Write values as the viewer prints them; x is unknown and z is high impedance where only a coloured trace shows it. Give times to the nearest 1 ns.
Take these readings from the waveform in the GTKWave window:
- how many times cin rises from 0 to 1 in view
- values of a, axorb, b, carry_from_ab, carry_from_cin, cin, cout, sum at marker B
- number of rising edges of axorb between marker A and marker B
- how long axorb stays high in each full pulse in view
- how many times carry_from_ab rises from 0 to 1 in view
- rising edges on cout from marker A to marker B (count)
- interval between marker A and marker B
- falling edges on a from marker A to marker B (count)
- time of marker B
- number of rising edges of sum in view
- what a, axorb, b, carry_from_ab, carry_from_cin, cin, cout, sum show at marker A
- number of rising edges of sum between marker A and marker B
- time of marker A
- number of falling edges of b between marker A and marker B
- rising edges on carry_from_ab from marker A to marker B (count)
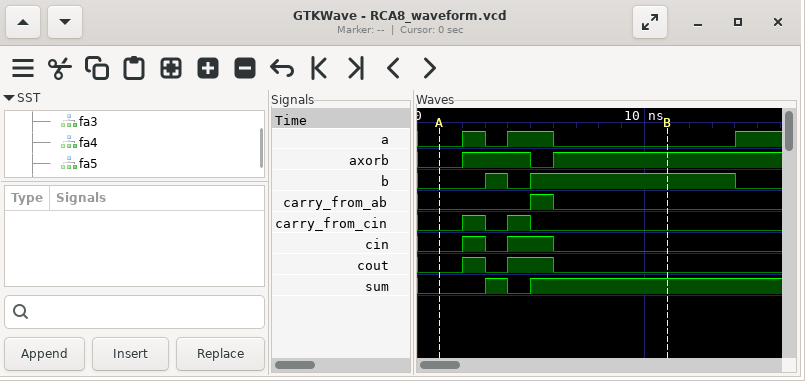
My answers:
2
a=0, axorb=1, b=1, carry_from_ab=0, carry_from_cin=0, cin=0, cout=0, sum=1
2
3 ns
1
2
10 ns
2
11 ns
2
a=0, axorb=0, b=0, carry_from_ab=0, carry_from_cin=0, cin=0, cout=0, sum=0
2
1 ns
1
1
